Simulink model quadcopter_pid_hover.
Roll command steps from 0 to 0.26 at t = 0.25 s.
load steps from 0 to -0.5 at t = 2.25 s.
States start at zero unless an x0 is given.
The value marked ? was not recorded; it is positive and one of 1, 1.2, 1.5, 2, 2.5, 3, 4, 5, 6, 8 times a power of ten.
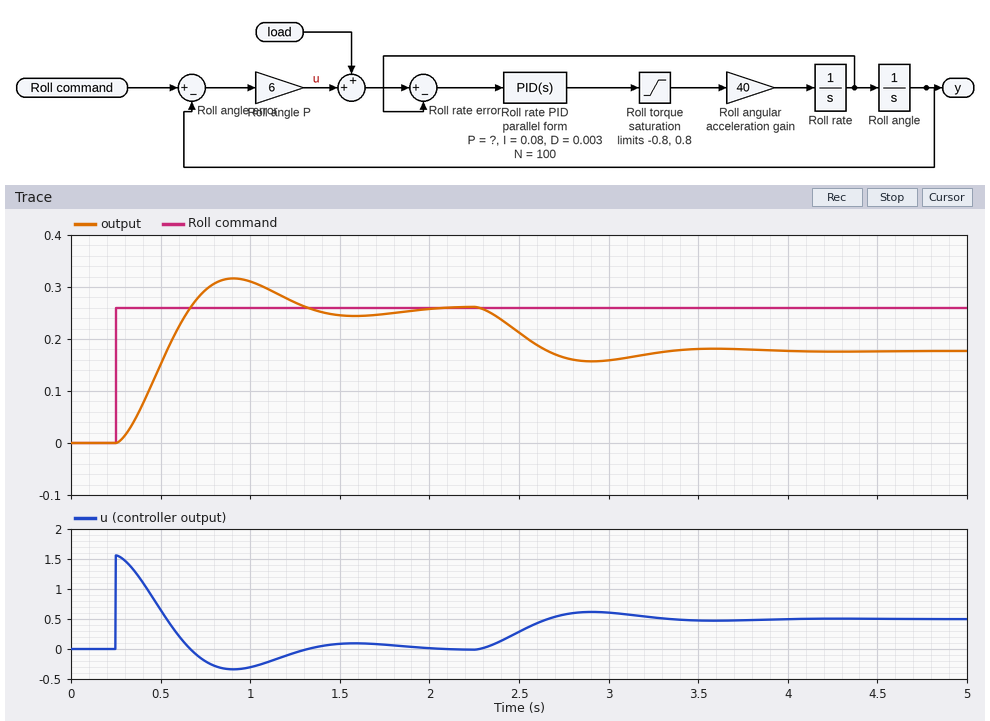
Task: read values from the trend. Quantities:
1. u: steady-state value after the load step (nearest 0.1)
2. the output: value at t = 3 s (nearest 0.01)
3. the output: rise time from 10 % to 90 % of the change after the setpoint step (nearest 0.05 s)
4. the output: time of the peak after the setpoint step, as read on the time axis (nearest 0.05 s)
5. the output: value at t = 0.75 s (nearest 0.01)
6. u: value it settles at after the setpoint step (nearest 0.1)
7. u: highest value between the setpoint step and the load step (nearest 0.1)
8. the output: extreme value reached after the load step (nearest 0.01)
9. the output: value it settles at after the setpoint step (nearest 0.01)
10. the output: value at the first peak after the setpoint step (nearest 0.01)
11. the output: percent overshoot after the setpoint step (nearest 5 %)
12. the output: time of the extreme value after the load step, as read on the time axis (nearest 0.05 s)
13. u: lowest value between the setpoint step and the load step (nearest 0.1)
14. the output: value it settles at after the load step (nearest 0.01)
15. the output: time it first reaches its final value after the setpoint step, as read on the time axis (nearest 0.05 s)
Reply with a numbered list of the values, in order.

1. 0.5
2. 0.16
3. 0.30 s
4. 0.90 s
5. 0.29
6. 0.0
7. 1.6
8. 0.16
9. 0.26
10. 0.32
11. 20 %
12. 2.90 s
13. -0.3
14. 0.18
15. 0.65 s
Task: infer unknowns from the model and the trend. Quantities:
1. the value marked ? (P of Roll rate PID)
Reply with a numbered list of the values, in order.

1. 0.12
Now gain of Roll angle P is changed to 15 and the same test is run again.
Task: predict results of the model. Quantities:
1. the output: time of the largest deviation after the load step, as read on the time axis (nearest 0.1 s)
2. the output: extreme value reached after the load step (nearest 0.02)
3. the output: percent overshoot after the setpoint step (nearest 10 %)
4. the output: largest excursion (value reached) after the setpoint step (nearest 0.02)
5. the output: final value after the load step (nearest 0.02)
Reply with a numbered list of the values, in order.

1. 2.6 s
2. 0.22
3. 30 %
4. 0.34
5. 0.22
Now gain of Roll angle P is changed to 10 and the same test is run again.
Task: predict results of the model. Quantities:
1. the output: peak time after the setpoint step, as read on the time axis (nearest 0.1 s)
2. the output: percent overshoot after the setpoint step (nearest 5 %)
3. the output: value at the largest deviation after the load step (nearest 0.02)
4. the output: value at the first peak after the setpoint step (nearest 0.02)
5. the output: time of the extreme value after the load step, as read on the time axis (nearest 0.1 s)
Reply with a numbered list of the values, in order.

1. 0.7 s
2. 30 %
3. 0.20
4. 0.34
5. 2.7 s
